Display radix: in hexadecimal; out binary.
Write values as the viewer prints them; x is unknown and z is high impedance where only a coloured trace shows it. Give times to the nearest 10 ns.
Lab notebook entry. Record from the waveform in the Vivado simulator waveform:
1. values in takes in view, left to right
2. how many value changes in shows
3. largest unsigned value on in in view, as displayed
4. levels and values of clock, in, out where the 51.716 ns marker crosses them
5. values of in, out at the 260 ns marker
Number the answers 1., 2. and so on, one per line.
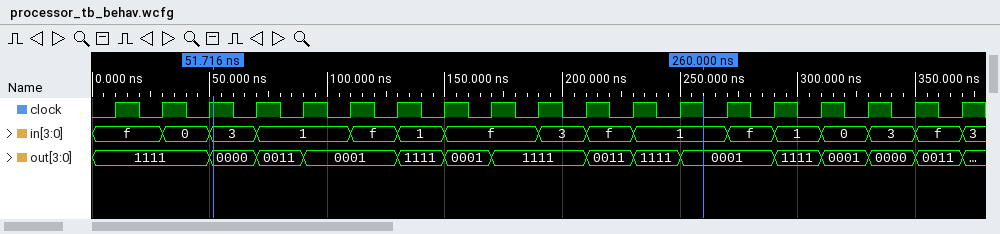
1. f, 0, 3, 1, f, 1, f, 3, f, 1, f, 1, 0, 3, f, 3
2. 15
3. f
4. clock=1, in=3, out=0000
5. in=1, out=0001
